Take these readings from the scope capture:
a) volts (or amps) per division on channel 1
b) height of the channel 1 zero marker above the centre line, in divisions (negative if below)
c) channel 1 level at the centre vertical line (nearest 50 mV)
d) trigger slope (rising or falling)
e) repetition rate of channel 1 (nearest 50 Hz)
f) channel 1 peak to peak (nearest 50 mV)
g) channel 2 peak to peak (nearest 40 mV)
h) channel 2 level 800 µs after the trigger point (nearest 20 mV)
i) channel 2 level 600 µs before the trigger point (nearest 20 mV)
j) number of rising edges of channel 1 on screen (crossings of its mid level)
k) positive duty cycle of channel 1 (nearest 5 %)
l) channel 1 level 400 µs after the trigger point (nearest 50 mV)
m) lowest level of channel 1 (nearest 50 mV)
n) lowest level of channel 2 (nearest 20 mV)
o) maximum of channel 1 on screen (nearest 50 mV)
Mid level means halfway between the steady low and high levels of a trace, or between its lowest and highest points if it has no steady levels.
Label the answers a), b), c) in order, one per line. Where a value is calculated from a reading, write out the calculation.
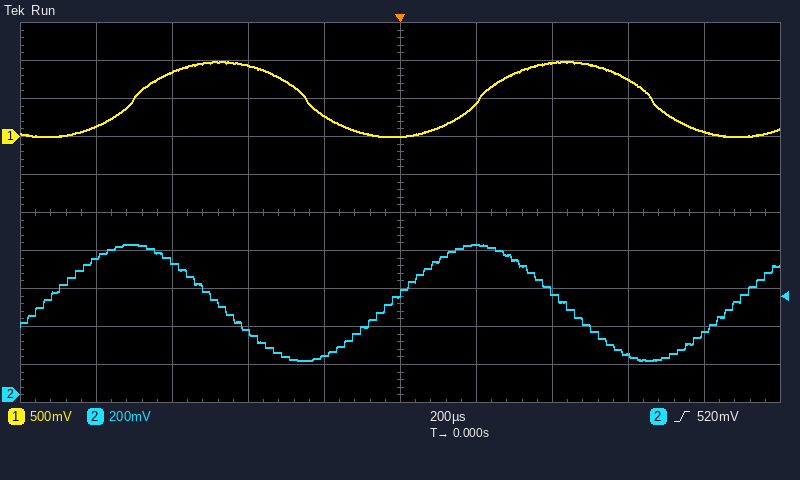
a) 500 mV
b) +2.0 div
c) 0 mV
d) rising
e) 1.10 kHz
f) 1.00 V − (0 mV) = 1.00 V
g) 600 mV
h) 320 mV
i) 700 mV
j) 2
k) 50 %
l) 950 mV
m) 0 mV
n) 180 mV
o) 1.00 V
